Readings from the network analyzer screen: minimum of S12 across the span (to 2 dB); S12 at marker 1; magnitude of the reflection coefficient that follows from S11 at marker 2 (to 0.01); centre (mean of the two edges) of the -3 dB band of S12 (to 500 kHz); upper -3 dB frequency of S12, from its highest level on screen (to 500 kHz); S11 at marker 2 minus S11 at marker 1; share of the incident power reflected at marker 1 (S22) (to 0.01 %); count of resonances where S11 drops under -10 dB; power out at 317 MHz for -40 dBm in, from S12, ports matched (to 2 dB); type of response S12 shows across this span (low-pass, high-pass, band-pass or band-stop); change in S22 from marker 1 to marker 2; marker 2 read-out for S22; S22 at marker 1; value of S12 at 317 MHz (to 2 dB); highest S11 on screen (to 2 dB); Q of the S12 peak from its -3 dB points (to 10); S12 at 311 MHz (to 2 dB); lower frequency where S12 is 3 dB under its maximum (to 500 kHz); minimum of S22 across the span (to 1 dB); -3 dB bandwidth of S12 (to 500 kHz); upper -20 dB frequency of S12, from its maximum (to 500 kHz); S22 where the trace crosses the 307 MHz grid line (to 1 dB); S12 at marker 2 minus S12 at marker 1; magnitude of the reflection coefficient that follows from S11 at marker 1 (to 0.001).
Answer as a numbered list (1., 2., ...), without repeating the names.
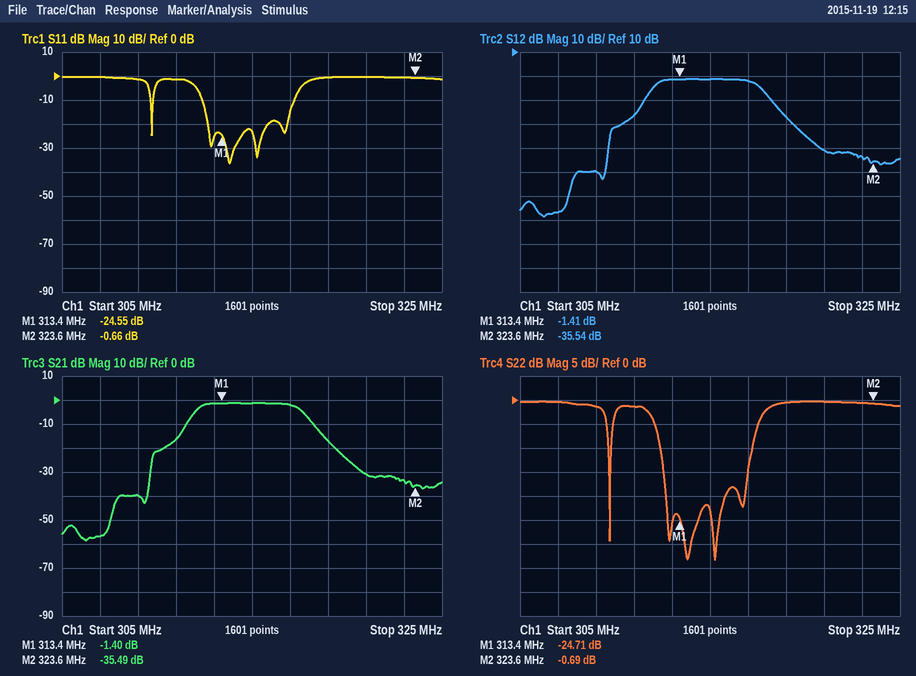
1. -58 dB
2. -1.41 dB
3. 0.93
4. 315.0 MHz
5. 317.5 MHz
6. 23.89 dB
7. 0.34 %
8. 5
9. -42 dBm
10. band-pass
11. 24.02 dB
12. -0.69 dB
13. -24.71 dB
14. -2 dB
15. 0 dB
16. 60
17. -16 dB
18. 312.0 MHz
19. -33 dB
20. 5.5 MHz
21. 319.5 MHz
22. 0 dB
23. -34.13 dB
24. 0.059
